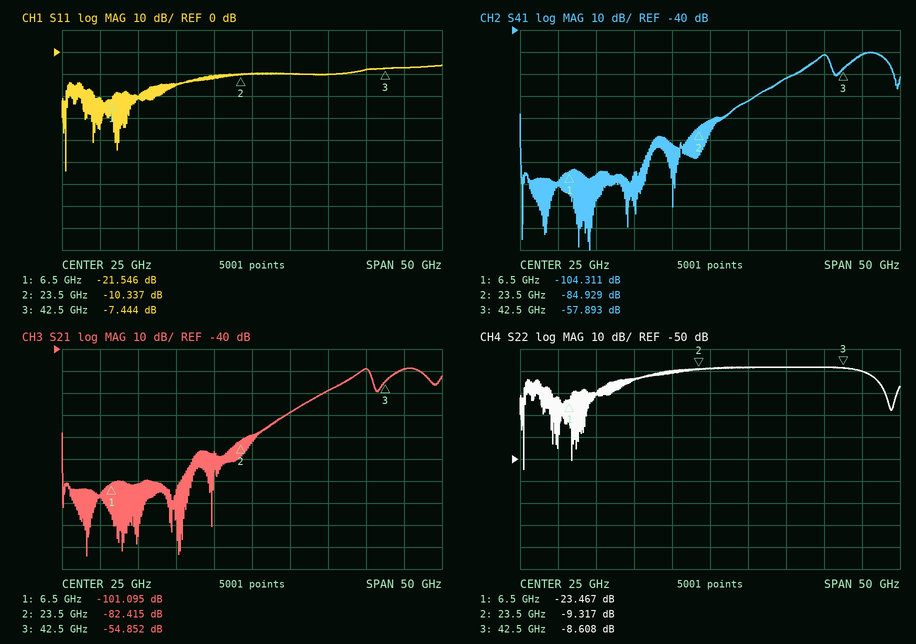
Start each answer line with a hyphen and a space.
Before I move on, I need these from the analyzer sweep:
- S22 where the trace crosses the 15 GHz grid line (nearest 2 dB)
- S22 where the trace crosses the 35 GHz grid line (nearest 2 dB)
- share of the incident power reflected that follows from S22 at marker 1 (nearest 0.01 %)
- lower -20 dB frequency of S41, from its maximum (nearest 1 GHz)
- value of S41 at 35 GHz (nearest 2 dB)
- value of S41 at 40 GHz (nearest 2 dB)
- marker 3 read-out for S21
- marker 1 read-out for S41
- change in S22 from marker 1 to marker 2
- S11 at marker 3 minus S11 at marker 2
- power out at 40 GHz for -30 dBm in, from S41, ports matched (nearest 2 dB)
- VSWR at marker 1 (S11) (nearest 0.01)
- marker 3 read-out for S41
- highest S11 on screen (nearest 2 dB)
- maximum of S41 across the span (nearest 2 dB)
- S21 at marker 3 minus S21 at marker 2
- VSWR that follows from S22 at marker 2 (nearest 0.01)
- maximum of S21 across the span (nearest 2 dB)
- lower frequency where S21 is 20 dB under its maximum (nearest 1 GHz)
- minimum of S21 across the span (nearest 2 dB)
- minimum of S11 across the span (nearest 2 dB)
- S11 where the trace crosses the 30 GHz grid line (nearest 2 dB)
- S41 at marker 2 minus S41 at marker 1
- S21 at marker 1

- -14 dB
- -8 dB
- 0.45 %
- 31 GHz
- -62 dB
- -52 dB
- -54.852 dB
- -104.311 dB
- 14.150 dB
- 2.893 dB
- -82 dBm
- 1.18
- -57.893 dB
- -6 dB
- -50 dB
- 27.563 dB
- 2.04
- -48 dB
- 30 GHz
- -134 dB
- -54 dB
- -10 dB
- 19.382 dB
- -101.095 dB
